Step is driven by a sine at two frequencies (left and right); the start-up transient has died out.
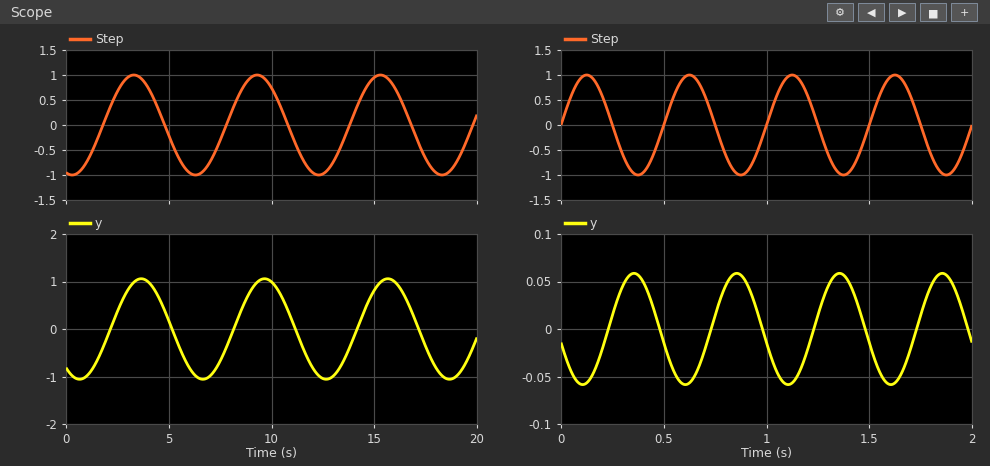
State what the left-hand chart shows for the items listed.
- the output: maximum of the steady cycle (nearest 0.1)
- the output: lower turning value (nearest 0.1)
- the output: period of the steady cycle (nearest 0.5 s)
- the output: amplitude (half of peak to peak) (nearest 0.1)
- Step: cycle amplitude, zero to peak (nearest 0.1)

1.1
-1.1
6.0 s
1.1
1.0
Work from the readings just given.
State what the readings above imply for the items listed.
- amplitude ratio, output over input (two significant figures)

1.1
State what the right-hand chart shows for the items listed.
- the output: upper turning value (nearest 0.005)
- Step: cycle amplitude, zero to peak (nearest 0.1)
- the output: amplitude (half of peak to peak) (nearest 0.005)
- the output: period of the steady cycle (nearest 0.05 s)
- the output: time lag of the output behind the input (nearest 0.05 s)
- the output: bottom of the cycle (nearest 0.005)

0.060
1.0
0.060
0.50 s
0.25 s
-0.060
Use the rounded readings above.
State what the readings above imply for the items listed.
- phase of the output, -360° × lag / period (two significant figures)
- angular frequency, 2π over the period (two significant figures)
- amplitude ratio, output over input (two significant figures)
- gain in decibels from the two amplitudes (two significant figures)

-180°
13 rad/s
0.060
-24 dB
